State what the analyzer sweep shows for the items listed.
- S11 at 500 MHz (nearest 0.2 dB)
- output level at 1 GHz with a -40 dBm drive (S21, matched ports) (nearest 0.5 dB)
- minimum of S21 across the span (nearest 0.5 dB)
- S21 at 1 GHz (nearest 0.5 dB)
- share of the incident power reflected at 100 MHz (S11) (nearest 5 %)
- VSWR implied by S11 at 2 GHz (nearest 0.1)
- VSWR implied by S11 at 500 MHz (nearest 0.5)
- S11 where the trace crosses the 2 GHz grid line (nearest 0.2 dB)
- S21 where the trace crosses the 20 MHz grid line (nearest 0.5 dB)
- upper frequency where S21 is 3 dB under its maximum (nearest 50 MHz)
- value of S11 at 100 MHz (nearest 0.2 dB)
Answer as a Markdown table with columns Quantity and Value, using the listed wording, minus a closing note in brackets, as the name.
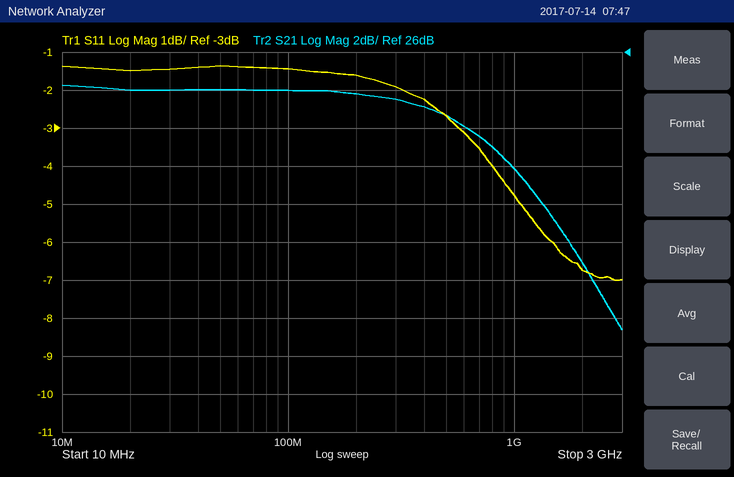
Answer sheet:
| Quantity | Value |
|---|---|
| S11 at 500 MHz | -2.6 dB |
| output level at 1 GHz with a -40 dBm drive (S21, matched ports) | -20.0 dBm |
| minimum of S21 across the span | 11.5 dB |
| S21 at 1 GHz | 20.0 dB |
| share of the incident power reflected at 100 MHz (S11) | 70 % |
| VSWR implied by S11 at 2 GHz | 2.7 |
| VSWR implied by S11 at 500 MHz | 6.5 |
| S11 where the trace crosses the 2 GHz grid line | -6.8 dB |
| S21 where the trace crosses the 20 MHz grid line | 24.0 dB |
| upper frequency where S21 is 3 dB under its maximum | 750 MHz |
| value of S11 at 100 MHz | -1.4 dB |
